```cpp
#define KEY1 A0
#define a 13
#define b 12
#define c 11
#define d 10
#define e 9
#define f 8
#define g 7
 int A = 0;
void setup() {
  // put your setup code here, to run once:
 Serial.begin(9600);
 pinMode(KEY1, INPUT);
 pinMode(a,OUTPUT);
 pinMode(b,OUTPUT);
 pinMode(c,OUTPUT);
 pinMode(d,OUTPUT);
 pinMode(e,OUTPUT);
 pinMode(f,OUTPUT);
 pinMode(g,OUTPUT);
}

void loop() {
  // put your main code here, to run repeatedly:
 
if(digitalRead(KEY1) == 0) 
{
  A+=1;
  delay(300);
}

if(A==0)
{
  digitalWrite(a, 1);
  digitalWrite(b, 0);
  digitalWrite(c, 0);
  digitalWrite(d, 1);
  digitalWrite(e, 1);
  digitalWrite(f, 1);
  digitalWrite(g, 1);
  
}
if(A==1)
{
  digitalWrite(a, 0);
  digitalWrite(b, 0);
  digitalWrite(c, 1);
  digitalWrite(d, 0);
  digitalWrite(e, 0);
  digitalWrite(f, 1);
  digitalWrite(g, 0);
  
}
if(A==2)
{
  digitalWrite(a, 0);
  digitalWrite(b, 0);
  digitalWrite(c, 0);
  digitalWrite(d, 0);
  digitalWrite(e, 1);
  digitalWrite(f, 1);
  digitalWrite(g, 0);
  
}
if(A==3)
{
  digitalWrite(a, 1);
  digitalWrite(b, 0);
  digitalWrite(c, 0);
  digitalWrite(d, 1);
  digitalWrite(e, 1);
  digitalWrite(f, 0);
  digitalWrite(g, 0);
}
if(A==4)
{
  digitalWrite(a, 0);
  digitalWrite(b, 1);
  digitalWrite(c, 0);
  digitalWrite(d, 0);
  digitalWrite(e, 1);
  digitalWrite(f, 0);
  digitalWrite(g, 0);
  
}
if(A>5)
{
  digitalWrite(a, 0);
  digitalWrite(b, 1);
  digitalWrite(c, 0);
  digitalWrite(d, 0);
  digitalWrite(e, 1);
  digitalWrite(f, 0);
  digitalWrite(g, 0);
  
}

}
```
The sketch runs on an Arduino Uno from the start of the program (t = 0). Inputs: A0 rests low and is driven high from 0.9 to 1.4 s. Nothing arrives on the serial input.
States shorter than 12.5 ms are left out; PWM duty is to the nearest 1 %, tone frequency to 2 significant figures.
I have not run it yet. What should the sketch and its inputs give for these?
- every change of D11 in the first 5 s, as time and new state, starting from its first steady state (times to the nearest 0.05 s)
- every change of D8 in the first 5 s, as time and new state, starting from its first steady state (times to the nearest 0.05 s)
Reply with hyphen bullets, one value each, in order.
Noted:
- 0 s low; 0.3 s high; 0.6 s low
- 0 s low; 0.3 s high; 0.9 s low
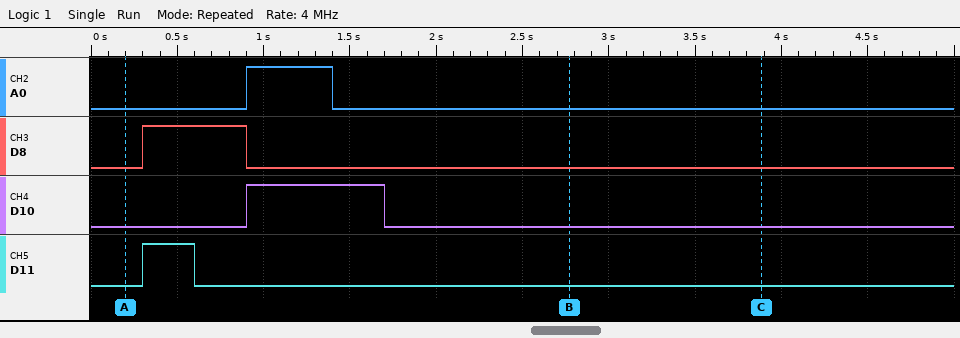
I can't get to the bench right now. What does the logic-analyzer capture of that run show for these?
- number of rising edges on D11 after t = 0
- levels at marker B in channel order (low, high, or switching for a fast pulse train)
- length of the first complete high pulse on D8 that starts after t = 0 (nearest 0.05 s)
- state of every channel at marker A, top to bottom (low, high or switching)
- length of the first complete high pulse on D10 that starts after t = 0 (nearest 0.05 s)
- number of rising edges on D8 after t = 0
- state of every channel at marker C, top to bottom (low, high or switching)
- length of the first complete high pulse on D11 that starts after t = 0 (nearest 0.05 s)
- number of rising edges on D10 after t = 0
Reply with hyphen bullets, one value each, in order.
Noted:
- 1
- A0 low, D8 low, D10 low, D11 low
- 0.60 s
- A0 low, D8 low, D10 low, D11 low
- 0.80 s
- 1
- A0 low, D8 low, D10 low, D11 low
- 0.30 s
- 1
